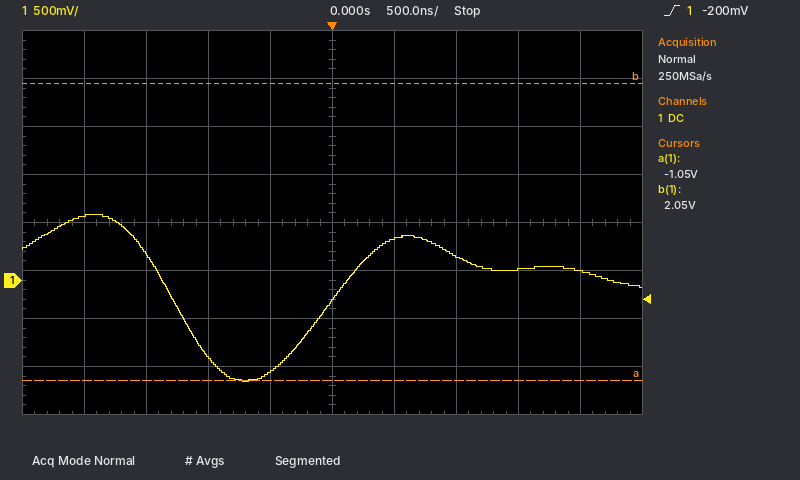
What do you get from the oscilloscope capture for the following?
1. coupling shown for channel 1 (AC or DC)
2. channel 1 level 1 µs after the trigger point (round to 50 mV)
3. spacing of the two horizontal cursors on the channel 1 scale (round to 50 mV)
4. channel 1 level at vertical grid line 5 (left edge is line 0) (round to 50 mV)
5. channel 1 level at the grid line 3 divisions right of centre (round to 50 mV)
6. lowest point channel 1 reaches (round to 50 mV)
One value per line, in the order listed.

DC
250 mV
3.10 V
-200 mV
100 mV
-1.05 V
